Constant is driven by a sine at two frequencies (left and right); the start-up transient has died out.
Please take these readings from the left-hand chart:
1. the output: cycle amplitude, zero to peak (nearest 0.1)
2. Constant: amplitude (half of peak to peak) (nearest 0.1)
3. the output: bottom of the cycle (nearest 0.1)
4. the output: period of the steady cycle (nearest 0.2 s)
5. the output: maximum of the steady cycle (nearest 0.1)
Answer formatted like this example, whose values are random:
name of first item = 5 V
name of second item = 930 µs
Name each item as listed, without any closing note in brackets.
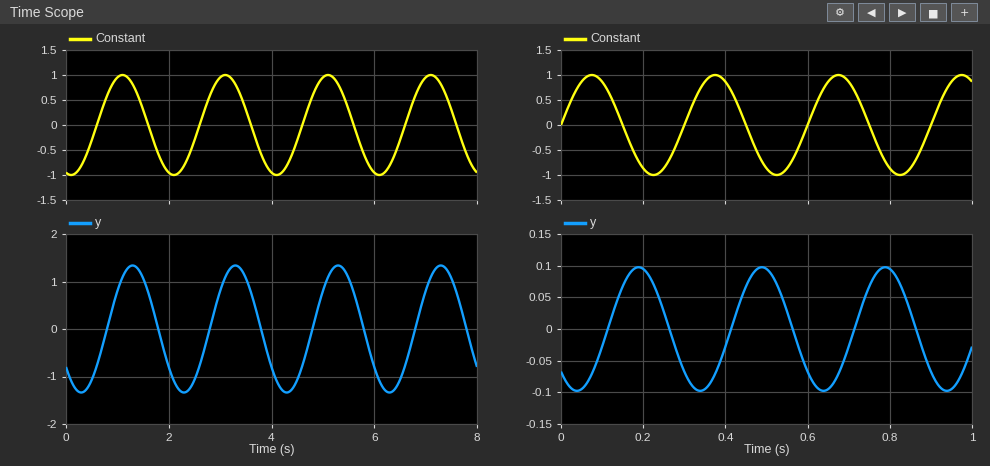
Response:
the output: cycle amplitude, zero to peak = 1.3
Constant: amplitude (half of peak to peak) = 1.0
the output: bottom of the cycle = -1.3
the output: period of the steady cycle = 2.0 s
the output: maximum of the steady cycle = 1.3
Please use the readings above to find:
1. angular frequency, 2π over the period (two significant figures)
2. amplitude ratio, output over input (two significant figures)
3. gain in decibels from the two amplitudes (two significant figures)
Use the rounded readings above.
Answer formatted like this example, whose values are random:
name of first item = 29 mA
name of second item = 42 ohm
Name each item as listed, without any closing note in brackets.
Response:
angular frequency, 2π over the period = 3.1 rad/s
amplitude ratio, output over input = 1.3
gain in decibels from the two amplitudes = 2.3 dB
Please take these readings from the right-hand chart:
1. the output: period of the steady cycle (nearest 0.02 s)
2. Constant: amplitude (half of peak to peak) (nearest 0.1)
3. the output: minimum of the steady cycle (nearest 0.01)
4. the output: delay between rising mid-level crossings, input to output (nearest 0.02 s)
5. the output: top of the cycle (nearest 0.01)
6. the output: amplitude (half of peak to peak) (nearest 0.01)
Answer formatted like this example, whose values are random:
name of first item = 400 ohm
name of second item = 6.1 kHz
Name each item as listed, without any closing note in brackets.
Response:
the output: period of the steady cycle = 0.30 s
Constant: amplitude (half of peak to peak) = 1.0
the output: minimum of the steady cycle = -0.10
the output: delay between rising mid-level crossings, input to output = 0.12 s
the output: top of the cycle = 0.10
the output: amplitude (half of peak to peak) = 0.10
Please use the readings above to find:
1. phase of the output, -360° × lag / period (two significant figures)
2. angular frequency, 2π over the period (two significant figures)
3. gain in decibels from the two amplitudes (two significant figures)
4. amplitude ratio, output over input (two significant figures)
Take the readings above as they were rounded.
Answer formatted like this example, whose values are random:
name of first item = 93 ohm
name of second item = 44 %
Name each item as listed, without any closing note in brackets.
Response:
phase of the output, -360° × lag / period = -140°
angular frequency, 2π over the period = 21 rad/s
gain in decibels from the two amplitudes = -20 dB
amplitude ratio, output over input = 0.10
